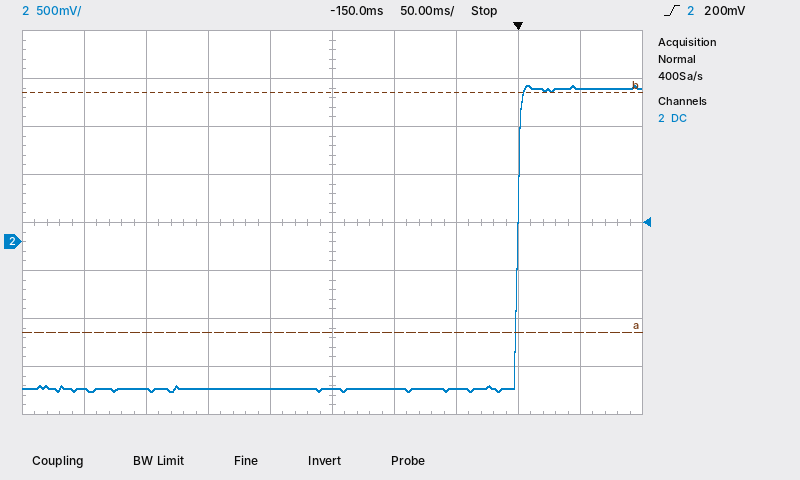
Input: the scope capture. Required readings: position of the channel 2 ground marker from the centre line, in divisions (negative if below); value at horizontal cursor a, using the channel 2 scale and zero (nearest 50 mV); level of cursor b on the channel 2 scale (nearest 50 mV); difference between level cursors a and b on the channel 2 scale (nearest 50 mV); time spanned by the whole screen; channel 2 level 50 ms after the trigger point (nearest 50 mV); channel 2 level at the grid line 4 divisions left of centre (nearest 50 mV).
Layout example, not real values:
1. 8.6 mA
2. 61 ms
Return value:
1. -0.4 div
2. -950 mV
3. 1.55 V
4. 2.50 V
5. 500 ms
6. 1.60 V
7. -1.55 V
